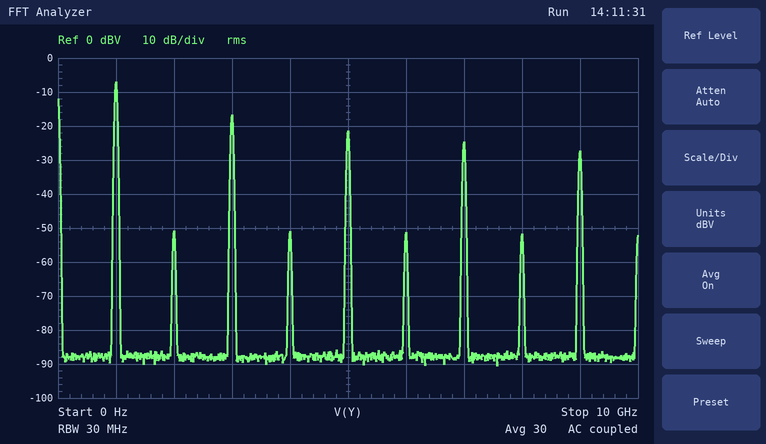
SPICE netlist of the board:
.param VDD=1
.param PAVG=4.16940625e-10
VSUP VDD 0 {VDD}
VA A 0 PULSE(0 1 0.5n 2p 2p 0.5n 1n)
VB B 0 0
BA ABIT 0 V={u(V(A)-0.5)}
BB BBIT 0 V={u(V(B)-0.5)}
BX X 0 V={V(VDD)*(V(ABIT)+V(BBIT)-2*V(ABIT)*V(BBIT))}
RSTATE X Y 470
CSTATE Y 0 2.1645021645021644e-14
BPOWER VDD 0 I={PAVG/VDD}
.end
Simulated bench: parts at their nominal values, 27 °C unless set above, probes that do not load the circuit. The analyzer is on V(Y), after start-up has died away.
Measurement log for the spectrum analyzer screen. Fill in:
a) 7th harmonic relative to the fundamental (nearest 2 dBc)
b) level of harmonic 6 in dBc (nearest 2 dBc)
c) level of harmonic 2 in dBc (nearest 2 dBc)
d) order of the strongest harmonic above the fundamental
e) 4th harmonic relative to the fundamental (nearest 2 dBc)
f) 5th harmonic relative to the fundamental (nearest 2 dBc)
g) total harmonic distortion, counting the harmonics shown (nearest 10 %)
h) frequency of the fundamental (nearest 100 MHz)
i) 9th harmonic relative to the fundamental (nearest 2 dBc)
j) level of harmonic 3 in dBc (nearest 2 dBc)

-18 dBc
-44 dBc
-44 dBc
3
-44 dBc
-14 dBc
40 %
1.0 GHz
-20 dBc
-10 dBc
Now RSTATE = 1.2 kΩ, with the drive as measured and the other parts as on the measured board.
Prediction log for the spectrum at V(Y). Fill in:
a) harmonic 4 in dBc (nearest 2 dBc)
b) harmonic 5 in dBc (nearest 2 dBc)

-46 dBc
-16 dBc
